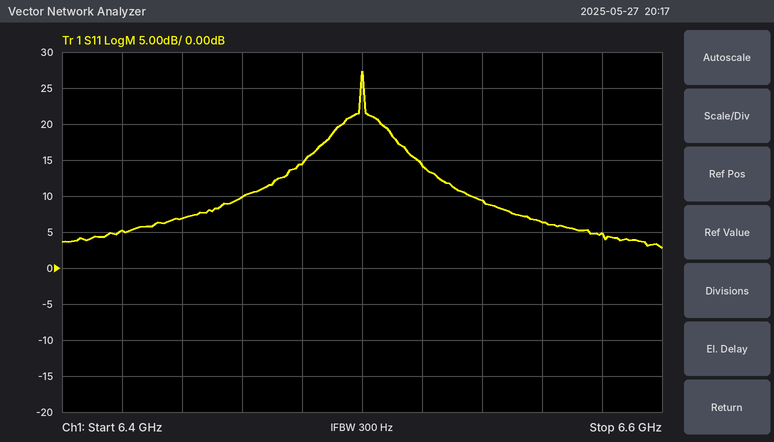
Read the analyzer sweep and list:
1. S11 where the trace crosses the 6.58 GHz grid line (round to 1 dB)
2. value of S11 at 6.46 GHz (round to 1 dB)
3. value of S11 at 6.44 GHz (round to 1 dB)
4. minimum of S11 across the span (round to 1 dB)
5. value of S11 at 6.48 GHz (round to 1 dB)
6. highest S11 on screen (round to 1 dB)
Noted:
5 dB
10 dB
7 dB
3 dB
14 dB
27 dB
